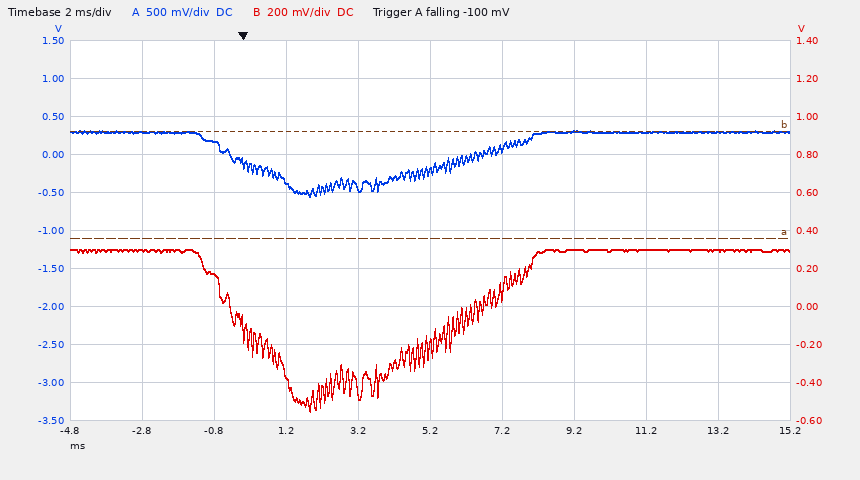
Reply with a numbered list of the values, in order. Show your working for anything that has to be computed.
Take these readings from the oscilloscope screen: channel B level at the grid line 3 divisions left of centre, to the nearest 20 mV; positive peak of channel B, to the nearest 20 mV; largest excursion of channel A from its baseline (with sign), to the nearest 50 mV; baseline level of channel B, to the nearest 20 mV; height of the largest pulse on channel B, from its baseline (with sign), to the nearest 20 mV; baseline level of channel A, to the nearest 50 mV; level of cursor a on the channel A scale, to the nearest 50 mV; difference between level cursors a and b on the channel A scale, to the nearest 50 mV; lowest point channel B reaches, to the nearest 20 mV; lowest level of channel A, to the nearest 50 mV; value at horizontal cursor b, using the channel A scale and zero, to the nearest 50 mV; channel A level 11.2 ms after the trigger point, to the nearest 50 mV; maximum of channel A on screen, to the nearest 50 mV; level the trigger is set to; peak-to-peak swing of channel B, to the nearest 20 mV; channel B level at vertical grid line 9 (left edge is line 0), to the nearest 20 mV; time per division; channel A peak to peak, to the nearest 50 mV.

1. 160 mV
2. 300 mV
3. -550 mV − (300 mV) = -850 mV
4. 300 mV
5. -560 mV − (300 mV) = -860 mV
6. 300 mV
7. -1.10 V
8. 1.40 V
9. -560 mV
10. -550 mV
11. 300 mV
12. 300 mV
13. 300 mV
14. -100 mV
15. 300 mV − (-560 mV) = 860 mV
16. 300 mV
17. 2 ms
18. 300 mV − (-550 mV) = 850 mV
